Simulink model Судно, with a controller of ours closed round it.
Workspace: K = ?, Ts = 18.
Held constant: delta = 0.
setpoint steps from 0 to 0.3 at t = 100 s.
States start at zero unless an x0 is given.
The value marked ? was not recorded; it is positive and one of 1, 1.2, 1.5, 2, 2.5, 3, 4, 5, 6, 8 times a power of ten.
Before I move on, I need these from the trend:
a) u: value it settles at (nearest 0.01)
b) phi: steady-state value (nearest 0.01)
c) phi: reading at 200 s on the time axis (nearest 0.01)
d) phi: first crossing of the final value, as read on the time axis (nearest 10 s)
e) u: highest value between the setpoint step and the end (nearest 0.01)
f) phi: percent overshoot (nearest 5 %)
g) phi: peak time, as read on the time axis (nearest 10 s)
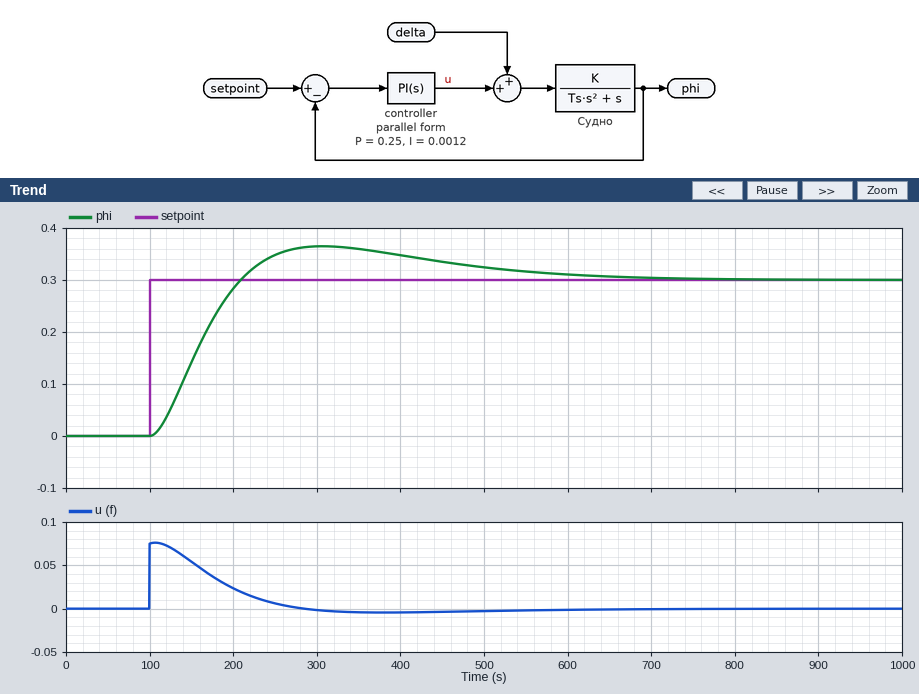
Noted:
0.00
0.30
0.28
210 s
0.08
20 %
310 s
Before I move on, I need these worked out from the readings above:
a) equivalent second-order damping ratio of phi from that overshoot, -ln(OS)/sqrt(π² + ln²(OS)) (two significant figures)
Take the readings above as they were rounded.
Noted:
0.46
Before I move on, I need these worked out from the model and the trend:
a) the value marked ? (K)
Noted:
0.06
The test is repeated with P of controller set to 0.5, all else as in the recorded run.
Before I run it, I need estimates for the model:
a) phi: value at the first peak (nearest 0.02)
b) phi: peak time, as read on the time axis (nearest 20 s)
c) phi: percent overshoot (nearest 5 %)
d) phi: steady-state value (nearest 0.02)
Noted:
0.34
200 s
15 %
0.30
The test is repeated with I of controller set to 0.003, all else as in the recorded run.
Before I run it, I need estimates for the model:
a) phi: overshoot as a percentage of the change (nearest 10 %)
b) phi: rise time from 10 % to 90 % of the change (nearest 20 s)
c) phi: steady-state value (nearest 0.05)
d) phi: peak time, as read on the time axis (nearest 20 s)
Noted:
40 %
60 s
0.30
260 s
